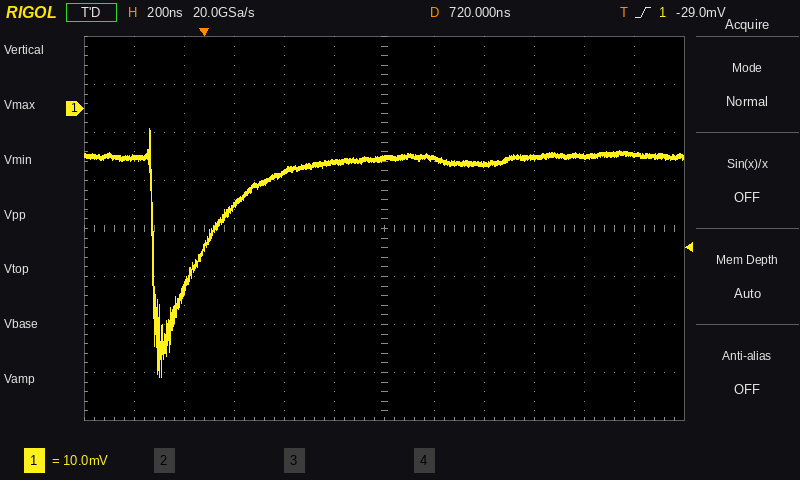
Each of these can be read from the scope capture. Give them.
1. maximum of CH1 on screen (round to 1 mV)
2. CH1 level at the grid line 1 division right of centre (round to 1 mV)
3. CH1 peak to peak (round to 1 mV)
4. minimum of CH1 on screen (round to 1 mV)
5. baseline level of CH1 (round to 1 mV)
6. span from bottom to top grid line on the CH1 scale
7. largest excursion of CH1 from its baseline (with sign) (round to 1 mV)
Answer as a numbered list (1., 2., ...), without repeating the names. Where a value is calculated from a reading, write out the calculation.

1. -4 mV
2. -10 mV
3. -4 mV − (-56 mV) = 52 mV
4. -56 mV
5. -10 mV
6. 80 mV
7. -56 mV − (-10 mV) = -46 mV
